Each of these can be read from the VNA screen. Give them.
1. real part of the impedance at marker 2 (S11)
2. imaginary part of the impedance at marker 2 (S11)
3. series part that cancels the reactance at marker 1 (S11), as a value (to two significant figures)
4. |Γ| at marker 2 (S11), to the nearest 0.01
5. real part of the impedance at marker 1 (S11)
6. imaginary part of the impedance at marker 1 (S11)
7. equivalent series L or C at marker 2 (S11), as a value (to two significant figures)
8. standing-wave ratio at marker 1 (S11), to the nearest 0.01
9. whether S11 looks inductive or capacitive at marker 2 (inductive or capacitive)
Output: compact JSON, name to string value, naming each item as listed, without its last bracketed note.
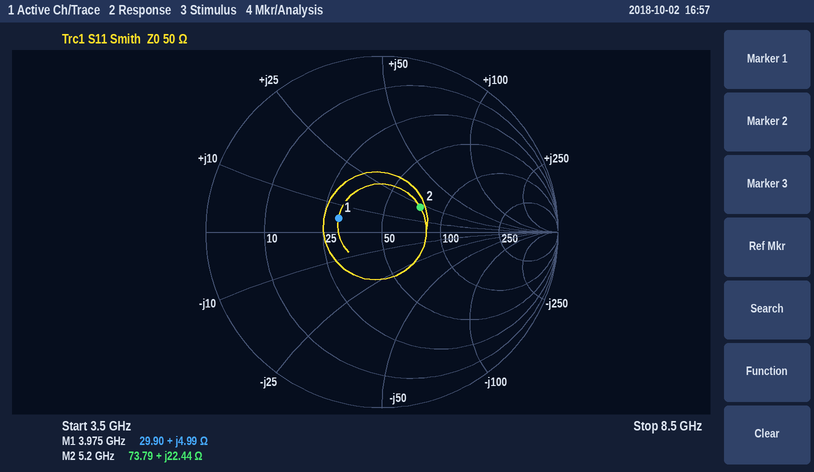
{"real part of the impedance at marker 2": "73.79 Ω", "imaginary part of the impedance at marker 2": "+22.44 Ω", "series part that cancels the reactance at marker 1 (S11), as a value": "8.0 pF", "|Γ| at marker 2 (S11), to the nearest 0.01": "0.26", "real part of the impedance at marker 1": "29.90 Ω", "imaginary part of the impedance at marker 1": "+4.99 Ω", "equivalent series L or C at marker 2 (S11), as a value": "690 pH", "standing-wave ratio at marker 1 (S11), to the nearest 0.01": "1.70", "whether S11 looks inductive or capacitive at marker 2": "inductive"}
